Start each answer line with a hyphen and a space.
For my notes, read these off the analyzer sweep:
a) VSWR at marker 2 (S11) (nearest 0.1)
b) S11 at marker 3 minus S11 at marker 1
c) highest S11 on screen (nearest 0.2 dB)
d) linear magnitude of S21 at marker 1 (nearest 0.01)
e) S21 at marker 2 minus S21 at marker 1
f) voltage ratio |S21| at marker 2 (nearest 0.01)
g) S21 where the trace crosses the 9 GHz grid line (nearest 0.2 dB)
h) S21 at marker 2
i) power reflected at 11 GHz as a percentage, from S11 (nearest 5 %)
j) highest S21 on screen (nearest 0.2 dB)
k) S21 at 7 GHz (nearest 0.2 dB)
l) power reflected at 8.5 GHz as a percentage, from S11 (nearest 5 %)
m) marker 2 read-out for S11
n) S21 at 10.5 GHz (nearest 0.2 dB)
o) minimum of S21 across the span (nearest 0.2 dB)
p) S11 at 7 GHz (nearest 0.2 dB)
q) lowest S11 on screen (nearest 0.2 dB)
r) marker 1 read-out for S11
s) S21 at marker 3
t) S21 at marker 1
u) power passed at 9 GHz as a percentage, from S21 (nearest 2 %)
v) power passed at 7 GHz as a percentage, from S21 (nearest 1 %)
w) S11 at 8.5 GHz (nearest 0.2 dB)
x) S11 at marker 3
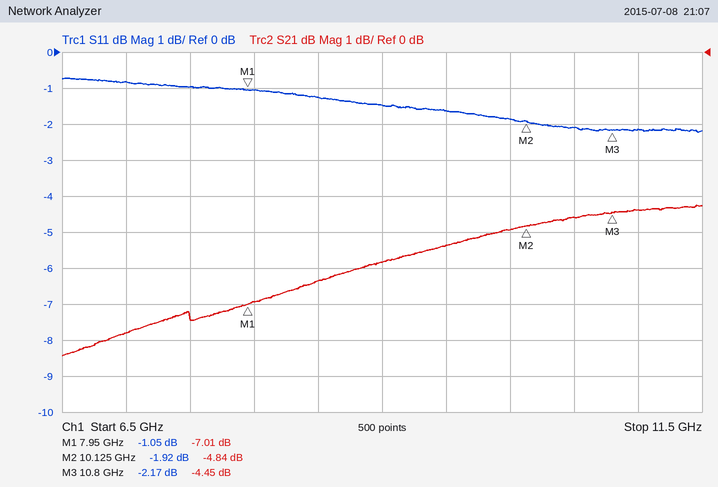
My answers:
- 9.1
- -1.12 dB
- -0.8 dB
- 0.45
- 2.17 dB
- 0.57
- -5.8 dB
- -4.84 dB
- 60 %
- -4.2 dB
- -7.8 dB
- 75 %
- -1.92 dB
- -4.6 dB
- -8.4 dB
- -0.8 dB
- -2.2 dB
- -1.05 dB
- -4.45 dB
- -7.01 dB
- 26 %
- 17 %
- -1.2 dB
- -2.17 dB
